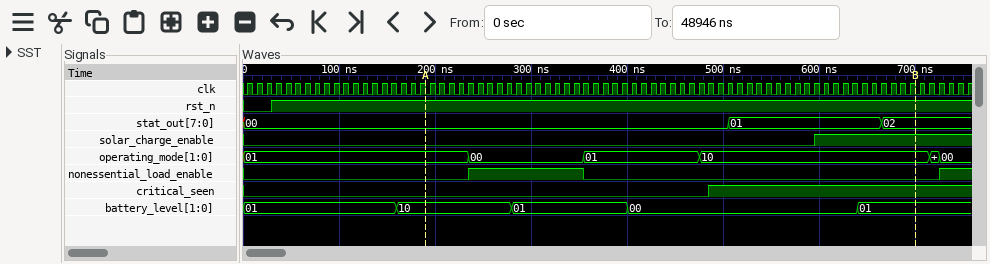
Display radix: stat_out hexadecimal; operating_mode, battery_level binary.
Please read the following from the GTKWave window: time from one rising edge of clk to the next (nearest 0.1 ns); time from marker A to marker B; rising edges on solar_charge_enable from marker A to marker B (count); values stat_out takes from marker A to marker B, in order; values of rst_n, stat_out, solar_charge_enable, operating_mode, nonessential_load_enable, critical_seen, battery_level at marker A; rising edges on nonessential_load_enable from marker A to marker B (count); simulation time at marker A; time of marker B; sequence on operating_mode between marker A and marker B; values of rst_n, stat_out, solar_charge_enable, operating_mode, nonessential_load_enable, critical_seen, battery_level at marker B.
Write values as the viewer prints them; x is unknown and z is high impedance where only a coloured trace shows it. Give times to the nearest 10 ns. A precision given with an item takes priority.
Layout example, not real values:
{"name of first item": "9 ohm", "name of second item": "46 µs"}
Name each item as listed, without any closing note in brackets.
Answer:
{"time from one rising edge of clk to the next": "10 ns", "time from marker A to marker B": "510 ns", "rising edges on solar_charge_enable from marker A to marker B": "1", "values stat_out takes from marker A to marker B, in order": "00, 01, 02", "values of rst_n, stat_out, solar_charge_enable, operating_mode, nonessential_load_enable, critical_seen, battery_level at marker A": "rst_n=1, stat_out=00, solar_charge_enable=0, operating_mode=01, nonessential_load_enable=0, critical_seen=0, battery_level=10", "rising edges on nonessential_load_enable from marker A to marker B": "1", "simulation time at marker A": "190 ns", "time of marker B": "700 ns", "sequence on operating_mode between marker A and marker B": "01, 00, 01, 10", "values of rst_n, stat_out, solar_charge_enable, operating_mode, nonessential_load_enable, critical_seen, battery_level at marker B": "rst_n=1, stat_out=02, solar_charge_enable=1, operating_mode=10, nonessential_load_enable=0, critical_seen=1, battery_level=01"}
